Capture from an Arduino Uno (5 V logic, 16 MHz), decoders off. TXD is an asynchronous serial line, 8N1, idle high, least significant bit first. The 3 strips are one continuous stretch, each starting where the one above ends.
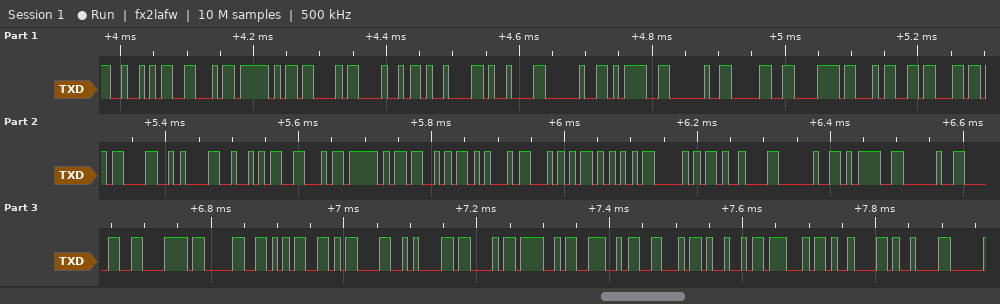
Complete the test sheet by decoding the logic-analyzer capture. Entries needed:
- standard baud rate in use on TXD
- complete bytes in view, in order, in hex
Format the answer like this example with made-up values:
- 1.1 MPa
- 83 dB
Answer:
- 115200 baud
- 52 46 5F 43 48 09 09 20 3D 20 30 78 34 63 0D 0A 52 46 5F 53 45 54 55 50 09 20 3D 20 30 78 30 35 0D 0A 43 4F 4E 46 49 47 09 09
